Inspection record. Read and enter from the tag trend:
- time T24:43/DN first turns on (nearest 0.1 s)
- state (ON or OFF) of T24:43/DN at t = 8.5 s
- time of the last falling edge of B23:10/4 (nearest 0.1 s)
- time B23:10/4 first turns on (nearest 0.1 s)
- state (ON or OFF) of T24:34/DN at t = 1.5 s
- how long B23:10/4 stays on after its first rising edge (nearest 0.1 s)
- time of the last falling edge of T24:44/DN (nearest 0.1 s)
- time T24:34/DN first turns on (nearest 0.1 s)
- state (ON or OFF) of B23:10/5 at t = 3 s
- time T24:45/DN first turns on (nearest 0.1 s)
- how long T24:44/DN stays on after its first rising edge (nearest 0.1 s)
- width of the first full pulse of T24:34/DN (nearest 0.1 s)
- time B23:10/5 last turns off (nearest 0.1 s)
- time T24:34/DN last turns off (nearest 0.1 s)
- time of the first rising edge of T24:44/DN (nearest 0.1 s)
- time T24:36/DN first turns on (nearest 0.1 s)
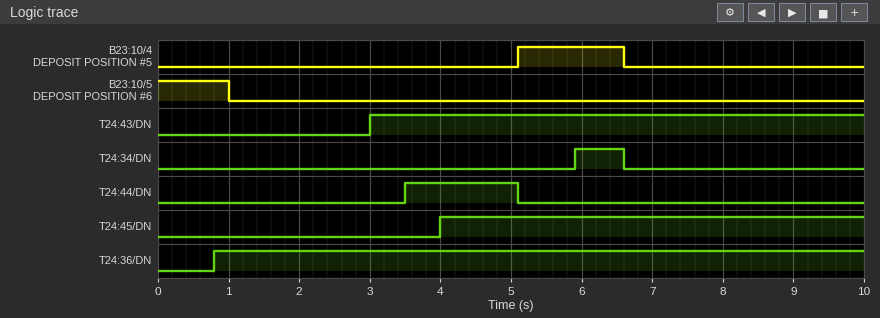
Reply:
3.0 s
ON
6.6 s
5.1 s
OFF
1.5 s
5.1 s
5.9 s
OFF
4.0 s
1.6 s
0.7 s
1.0 s
6.6 s
3.5 s
0.8 s
